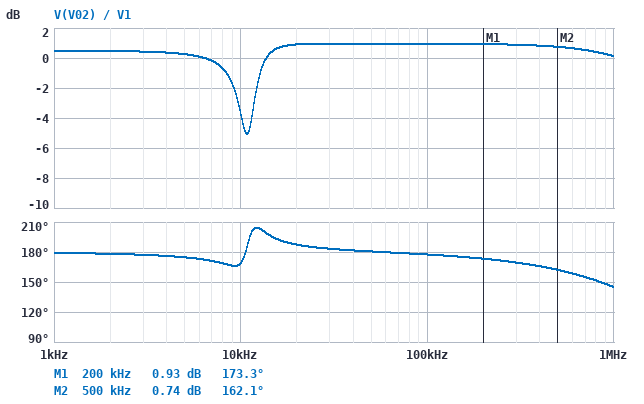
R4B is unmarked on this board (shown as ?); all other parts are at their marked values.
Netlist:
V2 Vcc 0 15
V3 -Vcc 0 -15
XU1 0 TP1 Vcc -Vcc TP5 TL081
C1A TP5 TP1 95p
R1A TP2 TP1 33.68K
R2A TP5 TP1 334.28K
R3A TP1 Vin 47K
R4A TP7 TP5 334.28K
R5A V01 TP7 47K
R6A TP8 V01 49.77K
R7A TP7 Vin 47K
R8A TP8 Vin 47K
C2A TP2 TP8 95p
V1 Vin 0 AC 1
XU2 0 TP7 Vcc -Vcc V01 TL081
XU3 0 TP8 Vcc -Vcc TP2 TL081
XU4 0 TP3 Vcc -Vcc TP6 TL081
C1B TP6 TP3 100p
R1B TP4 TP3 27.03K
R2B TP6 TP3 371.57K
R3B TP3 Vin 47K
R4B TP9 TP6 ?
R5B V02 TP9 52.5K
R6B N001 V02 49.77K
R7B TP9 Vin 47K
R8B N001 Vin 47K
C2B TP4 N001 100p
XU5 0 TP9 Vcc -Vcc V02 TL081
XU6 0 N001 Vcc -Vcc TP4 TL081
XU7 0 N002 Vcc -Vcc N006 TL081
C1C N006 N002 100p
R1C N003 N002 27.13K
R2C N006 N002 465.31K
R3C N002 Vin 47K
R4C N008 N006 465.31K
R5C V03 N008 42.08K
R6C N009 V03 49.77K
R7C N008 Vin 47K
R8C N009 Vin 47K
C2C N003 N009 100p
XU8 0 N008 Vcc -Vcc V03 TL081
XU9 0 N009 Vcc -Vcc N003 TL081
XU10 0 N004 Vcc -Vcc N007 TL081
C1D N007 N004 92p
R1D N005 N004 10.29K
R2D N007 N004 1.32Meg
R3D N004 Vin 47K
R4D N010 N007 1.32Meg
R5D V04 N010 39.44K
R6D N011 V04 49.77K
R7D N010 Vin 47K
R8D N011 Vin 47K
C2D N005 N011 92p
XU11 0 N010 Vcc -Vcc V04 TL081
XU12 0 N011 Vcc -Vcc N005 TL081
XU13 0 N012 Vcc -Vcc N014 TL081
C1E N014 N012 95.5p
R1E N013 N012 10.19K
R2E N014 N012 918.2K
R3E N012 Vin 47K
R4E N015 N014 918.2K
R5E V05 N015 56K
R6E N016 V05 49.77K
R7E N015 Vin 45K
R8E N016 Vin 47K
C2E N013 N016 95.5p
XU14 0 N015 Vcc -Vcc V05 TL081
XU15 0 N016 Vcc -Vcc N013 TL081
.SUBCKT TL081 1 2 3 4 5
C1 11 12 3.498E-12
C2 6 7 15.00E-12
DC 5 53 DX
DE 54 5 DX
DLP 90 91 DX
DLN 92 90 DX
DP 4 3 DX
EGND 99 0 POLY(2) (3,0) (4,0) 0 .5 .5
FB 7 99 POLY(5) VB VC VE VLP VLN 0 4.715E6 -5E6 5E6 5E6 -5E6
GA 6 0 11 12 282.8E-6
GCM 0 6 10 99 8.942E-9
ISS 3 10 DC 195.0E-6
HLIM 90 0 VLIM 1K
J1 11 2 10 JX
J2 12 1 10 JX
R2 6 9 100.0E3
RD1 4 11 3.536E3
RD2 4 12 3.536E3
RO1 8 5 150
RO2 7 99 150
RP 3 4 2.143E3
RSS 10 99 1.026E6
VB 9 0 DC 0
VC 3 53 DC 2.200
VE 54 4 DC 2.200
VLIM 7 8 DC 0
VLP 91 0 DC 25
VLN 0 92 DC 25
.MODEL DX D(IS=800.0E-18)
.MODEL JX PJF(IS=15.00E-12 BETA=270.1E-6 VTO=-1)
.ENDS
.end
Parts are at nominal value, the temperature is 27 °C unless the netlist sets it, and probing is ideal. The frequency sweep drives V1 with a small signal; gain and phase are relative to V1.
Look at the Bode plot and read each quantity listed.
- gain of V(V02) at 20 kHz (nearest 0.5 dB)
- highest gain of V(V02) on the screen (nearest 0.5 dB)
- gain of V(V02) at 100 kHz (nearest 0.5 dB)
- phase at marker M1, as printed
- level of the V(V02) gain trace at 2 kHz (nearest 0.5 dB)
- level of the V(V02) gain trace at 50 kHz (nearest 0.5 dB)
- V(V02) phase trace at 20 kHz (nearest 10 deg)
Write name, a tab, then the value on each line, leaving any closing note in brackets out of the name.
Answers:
gain of V(V02) at 20 kHz	1.0 dB
highest gain of V(V02) on the screen	1.0 dB
gain of V(V02) at 100 kHz	1.0 dB
phase at marker M1, as printed	173.3 deg
level of the V(V02) gain trace at 2 kHz	0.5 dB
level of the V(V02) gain trace at 50 kHz	1.0 dB
V(V02) phase trace at 20 kHz	190 deg
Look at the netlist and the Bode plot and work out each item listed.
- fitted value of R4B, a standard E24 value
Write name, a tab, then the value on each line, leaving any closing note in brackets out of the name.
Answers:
fitted value of R4B, a standard E24 value	750 kΩ
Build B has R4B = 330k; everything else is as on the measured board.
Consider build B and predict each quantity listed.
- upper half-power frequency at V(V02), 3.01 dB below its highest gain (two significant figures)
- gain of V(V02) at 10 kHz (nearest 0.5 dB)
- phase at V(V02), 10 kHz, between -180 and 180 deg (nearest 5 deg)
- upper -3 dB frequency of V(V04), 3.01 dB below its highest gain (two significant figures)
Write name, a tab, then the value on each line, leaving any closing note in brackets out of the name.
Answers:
upper half-power frequency at V(V02), 3.01 dB below its highest gain	1.9 MHz
gain of V(V02) at 10 kHz	0 dB
phase at V(V02), 10 kHz, between -180 and 180 deg	165 deg
upper -3 dB frequency of V(V04), 3.01 dB below its highest gain	13 kHz
